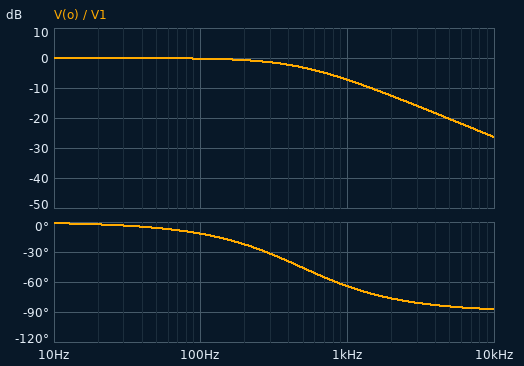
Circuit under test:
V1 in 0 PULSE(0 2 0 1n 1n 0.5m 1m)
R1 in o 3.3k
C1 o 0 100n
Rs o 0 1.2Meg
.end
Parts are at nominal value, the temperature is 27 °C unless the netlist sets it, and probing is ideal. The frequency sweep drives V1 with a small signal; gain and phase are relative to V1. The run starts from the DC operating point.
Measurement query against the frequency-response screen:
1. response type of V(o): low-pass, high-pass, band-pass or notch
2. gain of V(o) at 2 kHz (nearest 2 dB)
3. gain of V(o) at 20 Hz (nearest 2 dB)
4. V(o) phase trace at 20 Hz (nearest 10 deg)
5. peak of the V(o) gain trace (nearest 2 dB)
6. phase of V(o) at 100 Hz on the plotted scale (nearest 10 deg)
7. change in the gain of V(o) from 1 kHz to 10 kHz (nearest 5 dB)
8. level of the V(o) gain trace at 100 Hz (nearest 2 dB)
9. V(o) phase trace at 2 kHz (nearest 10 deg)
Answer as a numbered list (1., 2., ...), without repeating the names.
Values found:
1. low-pass
2. -12 dB
3. 0 dB
4. 0 deg
5. 0 dB
6. -10 deg
7. -20 dB
8. 0 dB
9. -80 deg
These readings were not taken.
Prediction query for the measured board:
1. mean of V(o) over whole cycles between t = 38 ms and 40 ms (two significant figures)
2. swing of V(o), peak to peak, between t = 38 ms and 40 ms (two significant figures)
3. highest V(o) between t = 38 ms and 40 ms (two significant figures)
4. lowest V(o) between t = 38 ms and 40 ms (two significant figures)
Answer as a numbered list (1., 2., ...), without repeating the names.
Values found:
1. 1.0 V
2. 1.3 V
3. 1.6 V
4. 360 mV
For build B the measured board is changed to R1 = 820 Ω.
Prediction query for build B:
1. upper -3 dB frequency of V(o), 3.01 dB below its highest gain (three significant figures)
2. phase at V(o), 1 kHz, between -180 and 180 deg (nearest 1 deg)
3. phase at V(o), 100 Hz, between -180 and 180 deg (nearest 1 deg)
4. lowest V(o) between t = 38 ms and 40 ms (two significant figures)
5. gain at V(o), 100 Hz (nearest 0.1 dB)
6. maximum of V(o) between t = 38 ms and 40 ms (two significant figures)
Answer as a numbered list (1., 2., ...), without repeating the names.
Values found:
1. 1.94 kHz
2. -27 deg
3. -3 deg
4. 4.5 mV
5. 0 dB
6. 2.0 V
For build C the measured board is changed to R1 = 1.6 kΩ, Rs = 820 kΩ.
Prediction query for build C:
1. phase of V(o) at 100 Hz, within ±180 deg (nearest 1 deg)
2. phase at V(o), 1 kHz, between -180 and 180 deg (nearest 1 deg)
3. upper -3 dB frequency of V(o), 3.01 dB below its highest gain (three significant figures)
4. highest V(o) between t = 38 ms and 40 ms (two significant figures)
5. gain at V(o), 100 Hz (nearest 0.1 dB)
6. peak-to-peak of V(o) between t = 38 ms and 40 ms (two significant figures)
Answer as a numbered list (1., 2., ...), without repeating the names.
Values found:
1. -6 deg
2. -45 deg
3. 997 Hz
4. 1.9 V
5. -0.1 dB
6. 1.8 V
